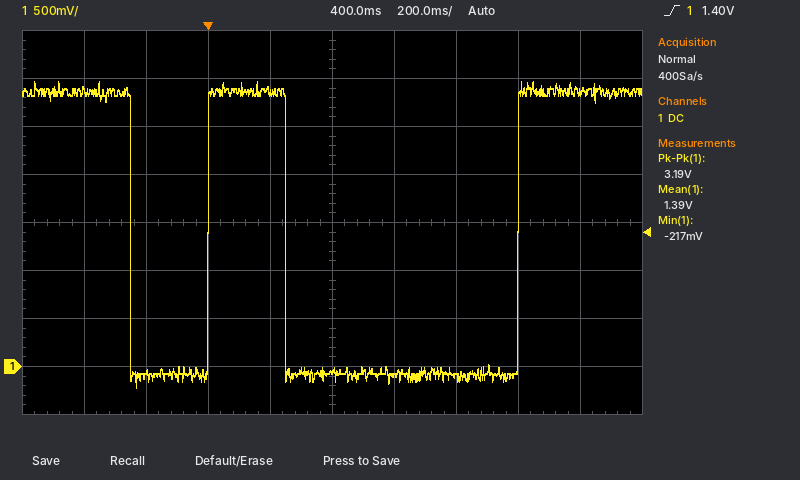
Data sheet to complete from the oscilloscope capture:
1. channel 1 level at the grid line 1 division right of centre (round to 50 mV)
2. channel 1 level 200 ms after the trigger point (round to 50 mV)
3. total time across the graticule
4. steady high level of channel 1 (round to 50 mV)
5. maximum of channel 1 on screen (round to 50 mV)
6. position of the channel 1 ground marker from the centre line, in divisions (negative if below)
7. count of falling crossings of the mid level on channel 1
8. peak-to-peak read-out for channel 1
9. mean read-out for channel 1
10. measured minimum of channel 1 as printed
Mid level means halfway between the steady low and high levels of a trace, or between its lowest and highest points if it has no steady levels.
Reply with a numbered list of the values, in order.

1. -100 mV
2. 2.85 V
3. 2 s
4. 2.85 V
5. 2.95 V
6. -3.0 div
7. 2
8. 3.19 V
9. 1.39 V
10. -217 mV
